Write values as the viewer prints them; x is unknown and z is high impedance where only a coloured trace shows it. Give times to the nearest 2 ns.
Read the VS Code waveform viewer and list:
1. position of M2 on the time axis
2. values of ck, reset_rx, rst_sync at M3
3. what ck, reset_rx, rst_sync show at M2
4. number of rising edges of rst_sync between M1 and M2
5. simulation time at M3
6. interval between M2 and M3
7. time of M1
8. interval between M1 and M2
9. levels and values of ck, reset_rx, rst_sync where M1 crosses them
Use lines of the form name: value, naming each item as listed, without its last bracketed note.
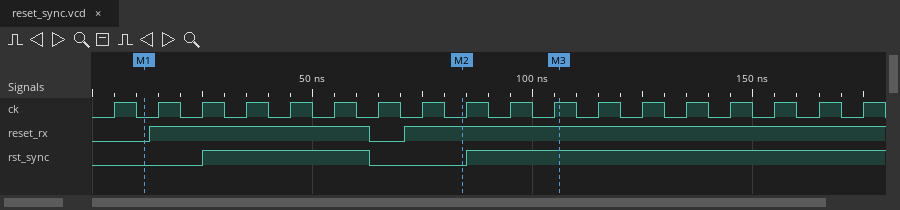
position of M2 on the time axis: 84 ns
values of ck, reset_rx, rst_sync at M3: ck=1, reset_rx=1, rst_sync=1
what ck, reset_rx, rst_sync show at M2: ck=0, reset_rx=1, rst_sync=0
number of rising edges of rst_sync between M1 and M2: 1
simulation time at M3: 106 ns
interval between M2 and M3: 22 ns
time of M1: 12 ns
interval between M1 and M2: 72 ns
levels and values of ck, reset_rx, rst_sync where M1 crosses them: ck=0, reset_rx=0, rst_sync=0
